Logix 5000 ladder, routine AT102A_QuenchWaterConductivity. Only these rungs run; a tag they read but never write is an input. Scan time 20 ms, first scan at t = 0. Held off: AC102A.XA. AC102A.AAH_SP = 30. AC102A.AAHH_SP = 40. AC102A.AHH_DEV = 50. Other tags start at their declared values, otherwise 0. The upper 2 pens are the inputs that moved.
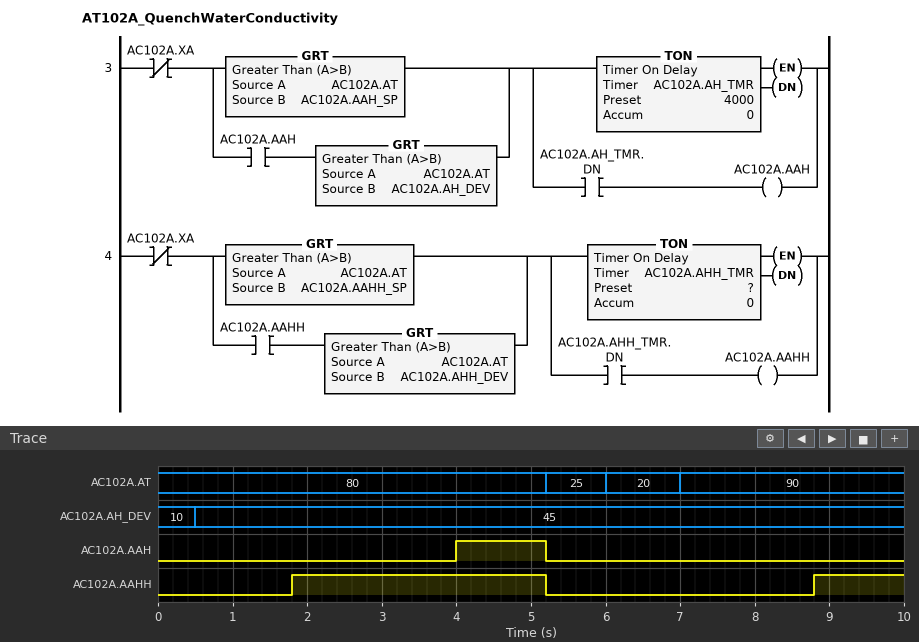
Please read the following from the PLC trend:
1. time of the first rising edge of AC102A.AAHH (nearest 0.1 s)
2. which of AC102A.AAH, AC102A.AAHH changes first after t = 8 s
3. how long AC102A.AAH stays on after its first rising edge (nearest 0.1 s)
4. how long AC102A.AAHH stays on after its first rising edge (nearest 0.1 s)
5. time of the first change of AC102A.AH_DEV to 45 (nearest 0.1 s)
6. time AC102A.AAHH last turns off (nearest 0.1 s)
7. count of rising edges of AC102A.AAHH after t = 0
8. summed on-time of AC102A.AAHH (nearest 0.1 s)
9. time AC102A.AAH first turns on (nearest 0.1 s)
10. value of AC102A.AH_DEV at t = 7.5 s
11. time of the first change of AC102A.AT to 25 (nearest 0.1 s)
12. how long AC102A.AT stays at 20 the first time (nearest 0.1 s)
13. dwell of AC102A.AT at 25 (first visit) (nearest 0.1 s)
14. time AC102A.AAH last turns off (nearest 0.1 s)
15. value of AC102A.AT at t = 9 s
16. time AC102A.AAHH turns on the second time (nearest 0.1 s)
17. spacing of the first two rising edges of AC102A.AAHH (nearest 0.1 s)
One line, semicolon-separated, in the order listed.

1.8 s; AC102A.AAHH; 1.2 s; 3.4 s; 0.5 s; 5.2 s; 2; 4.6 s; 4.0 s; 45; 5.2 s; 1.0 s; 0.8 s; 5.2 s; 90; 8.8 s; 7.0 s
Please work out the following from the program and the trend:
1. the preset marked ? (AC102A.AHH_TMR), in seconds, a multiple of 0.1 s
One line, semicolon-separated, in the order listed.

1.8 s
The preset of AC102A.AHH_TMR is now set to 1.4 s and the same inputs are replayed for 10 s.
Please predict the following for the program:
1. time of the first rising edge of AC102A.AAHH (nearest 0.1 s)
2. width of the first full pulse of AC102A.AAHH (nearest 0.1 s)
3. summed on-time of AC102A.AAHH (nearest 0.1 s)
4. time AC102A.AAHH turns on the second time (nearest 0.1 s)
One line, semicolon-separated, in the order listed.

1.4 s; 3.8 s; 5.4 s; 8.4 s
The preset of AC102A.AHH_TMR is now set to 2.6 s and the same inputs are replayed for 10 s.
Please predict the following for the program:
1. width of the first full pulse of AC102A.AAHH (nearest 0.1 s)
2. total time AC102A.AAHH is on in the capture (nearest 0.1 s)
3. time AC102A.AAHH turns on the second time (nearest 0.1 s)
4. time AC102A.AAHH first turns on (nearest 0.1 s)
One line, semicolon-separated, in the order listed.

2.6 s; 3.0 s; 9.6 s; 2.6 s
